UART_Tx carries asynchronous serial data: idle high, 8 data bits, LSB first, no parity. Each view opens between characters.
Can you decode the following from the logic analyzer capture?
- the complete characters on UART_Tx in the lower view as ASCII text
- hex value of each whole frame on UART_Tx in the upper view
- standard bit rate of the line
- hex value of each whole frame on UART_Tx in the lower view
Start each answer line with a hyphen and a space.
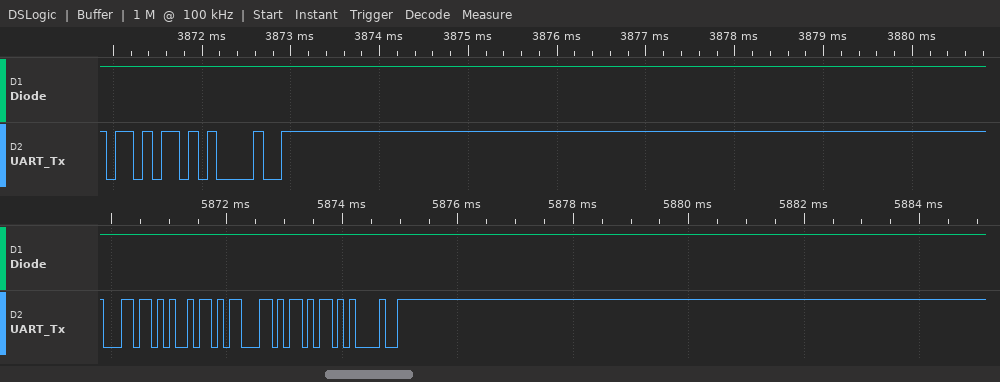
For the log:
- "lick!"
- 6B, 21
- 9600 baud
- 6C, 69, 63, 6B, 21
